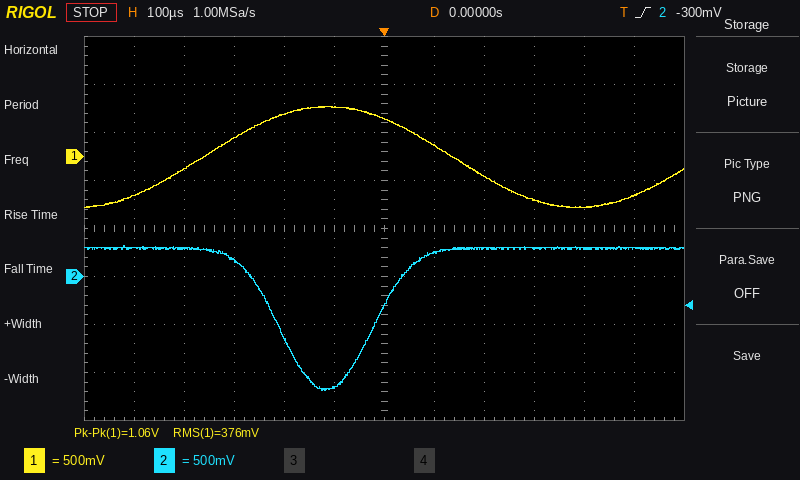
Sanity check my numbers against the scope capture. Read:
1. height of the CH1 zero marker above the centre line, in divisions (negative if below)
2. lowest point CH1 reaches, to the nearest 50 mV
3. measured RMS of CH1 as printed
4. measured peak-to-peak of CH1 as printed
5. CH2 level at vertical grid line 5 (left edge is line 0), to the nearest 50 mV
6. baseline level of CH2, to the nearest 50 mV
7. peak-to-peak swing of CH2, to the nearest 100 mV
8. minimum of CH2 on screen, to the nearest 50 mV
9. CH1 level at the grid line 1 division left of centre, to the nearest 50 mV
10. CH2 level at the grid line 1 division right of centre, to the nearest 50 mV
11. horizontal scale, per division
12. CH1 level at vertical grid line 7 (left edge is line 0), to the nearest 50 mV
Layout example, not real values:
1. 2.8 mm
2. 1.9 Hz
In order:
1. +1.5 div
2. -550 mV
3. 376 mV
4. 1.06 V
5. -1.15 V
6. 300 mV
7. 1.50 V
8. -1.20 V
9. 500 mV
10. 250 mV
11. 100 µs
12. 100 mV
